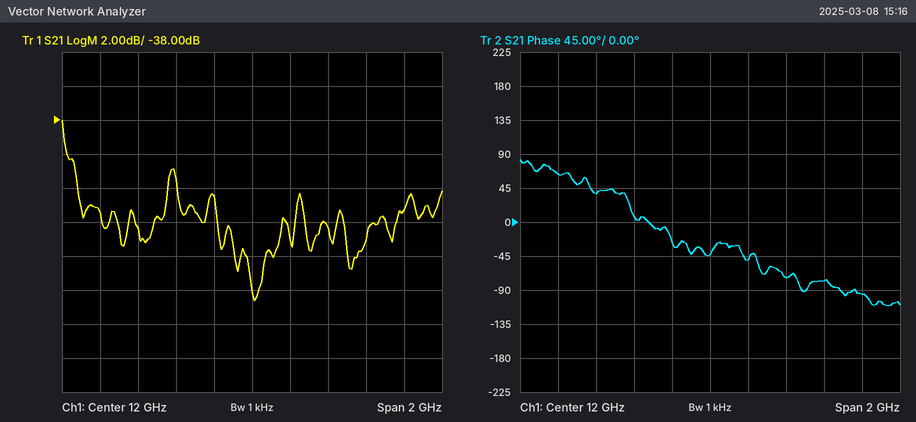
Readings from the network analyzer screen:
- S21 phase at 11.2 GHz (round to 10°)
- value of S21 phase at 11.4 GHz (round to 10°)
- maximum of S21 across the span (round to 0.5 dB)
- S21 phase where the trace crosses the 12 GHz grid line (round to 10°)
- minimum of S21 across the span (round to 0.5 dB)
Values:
60°
40°
-38.0 dB
-40°
-48.5 dB
